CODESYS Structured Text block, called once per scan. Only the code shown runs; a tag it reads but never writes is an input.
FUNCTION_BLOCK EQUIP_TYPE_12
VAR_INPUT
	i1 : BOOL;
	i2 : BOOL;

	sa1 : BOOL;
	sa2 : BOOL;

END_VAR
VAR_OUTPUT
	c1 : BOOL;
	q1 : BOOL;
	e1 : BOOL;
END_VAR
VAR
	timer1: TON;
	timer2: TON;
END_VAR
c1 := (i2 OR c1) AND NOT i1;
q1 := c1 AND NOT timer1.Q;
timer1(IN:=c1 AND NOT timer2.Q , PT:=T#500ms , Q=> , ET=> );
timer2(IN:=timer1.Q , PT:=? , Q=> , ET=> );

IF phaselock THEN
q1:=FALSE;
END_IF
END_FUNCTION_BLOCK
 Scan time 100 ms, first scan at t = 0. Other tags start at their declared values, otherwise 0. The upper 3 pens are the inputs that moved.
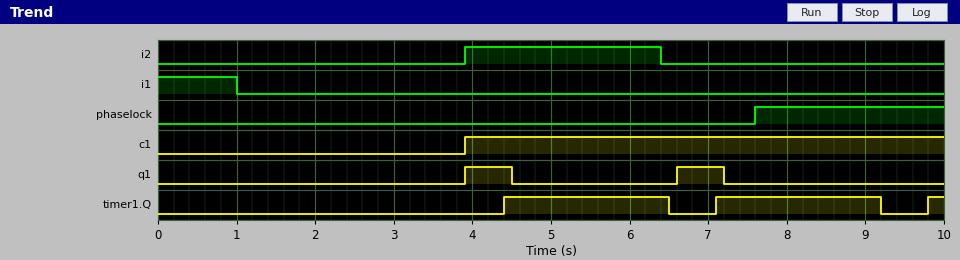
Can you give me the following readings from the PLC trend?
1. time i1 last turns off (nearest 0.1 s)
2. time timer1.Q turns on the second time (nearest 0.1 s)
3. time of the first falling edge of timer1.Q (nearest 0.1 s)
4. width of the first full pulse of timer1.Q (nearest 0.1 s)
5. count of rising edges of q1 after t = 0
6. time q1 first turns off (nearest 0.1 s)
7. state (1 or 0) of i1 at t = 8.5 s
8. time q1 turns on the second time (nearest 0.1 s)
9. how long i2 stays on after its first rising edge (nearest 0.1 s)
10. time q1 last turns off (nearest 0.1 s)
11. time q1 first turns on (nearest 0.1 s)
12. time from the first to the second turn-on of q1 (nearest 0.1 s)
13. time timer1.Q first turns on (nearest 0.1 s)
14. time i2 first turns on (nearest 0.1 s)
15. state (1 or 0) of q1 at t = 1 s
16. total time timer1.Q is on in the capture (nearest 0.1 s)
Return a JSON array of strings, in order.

["1.0 s", "7.1 s", "6.5 s", "2.1 s", "2", "4.5 s", "0", "6.6 s", "2.5 s", "7.2 s", "3.9 s", "2.7 s", "4.4 s", "3.9 s", "0", "4.4 s"]
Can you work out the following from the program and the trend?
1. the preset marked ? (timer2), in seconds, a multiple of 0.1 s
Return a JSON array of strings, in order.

["2.0 s"]
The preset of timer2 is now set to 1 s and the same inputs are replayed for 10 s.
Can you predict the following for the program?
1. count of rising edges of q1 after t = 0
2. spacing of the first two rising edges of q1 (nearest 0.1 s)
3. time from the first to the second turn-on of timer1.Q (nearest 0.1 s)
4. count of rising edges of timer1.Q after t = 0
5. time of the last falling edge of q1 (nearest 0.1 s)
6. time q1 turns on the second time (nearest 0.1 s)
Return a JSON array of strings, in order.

["3", "1.7 s", "1.7 s", "4", "7.6 s", "5.6 s"]
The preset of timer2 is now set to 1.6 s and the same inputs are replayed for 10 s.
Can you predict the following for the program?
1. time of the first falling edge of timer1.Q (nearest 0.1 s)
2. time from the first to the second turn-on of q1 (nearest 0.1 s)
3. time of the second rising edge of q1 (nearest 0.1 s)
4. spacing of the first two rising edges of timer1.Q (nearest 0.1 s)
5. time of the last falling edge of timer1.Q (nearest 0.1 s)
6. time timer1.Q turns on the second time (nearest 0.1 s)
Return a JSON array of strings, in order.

["6.1 s", "2.3 s", "6.2 s", "2.3 s", "8.4 s", "6.7 s"]
